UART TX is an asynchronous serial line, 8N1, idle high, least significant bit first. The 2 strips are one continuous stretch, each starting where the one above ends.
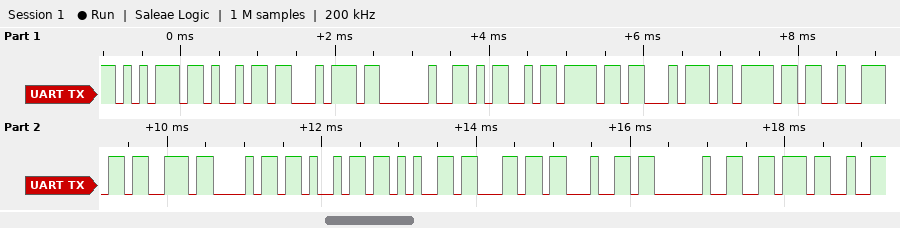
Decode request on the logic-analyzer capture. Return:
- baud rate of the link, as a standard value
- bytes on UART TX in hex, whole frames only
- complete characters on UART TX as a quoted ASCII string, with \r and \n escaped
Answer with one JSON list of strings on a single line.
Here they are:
["9600 baud", "0x75 0x69 0x74 0x20 0x4D 0x6F 0x74 0x6F 0x72 0x73 0x68 0x69 0x65 0x6C 0x64 0x20 0x76", "\"uit Motorshield v\""]
